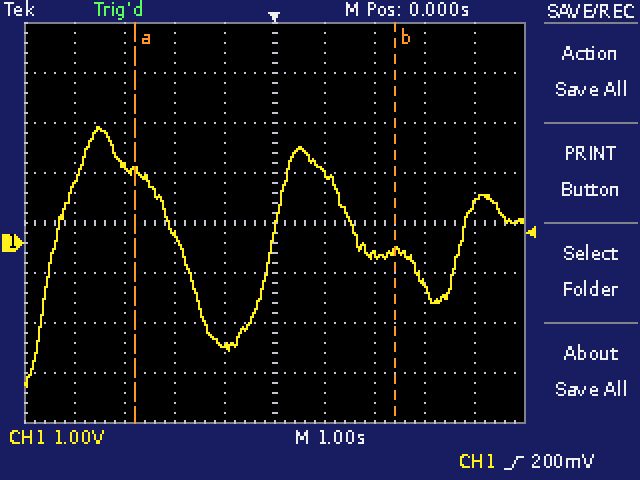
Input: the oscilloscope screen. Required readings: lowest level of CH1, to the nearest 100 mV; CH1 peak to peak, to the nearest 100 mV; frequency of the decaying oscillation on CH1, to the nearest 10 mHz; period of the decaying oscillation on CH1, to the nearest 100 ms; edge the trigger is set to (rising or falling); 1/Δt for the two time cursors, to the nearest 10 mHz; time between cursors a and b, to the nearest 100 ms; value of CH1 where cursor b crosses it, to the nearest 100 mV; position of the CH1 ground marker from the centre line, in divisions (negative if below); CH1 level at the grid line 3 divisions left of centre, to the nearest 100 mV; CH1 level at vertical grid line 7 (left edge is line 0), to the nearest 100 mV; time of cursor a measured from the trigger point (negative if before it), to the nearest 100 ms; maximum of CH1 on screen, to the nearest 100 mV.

-2.9 V
5.2 V
260 mHz
3.8 s
rising
190 mHz
5.2 s
-200 mV
-0.4 div
1.5 V
-200 mV
-2.8 s
2.3 V
